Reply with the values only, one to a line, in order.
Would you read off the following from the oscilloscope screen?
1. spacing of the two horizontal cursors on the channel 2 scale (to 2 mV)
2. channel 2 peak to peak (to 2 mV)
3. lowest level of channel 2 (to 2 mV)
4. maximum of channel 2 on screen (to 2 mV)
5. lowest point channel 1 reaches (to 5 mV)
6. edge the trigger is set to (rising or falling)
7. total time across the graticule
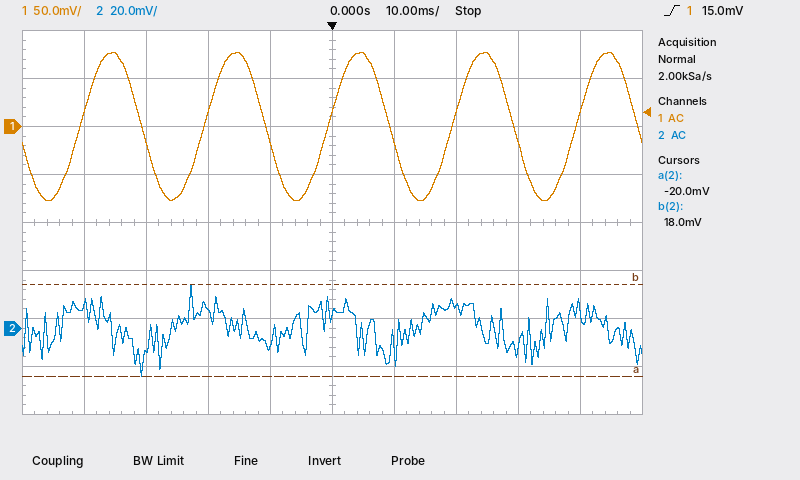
38 mV
38 mV
-20 mV
18 mV
-75 mV
rising
100 ms
